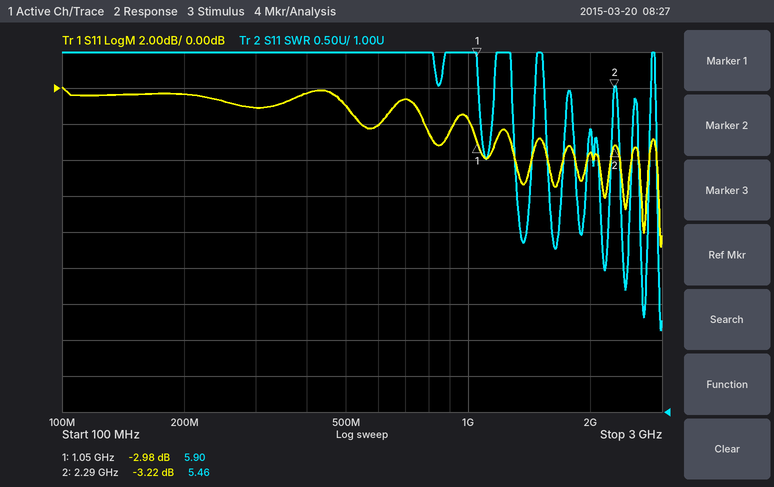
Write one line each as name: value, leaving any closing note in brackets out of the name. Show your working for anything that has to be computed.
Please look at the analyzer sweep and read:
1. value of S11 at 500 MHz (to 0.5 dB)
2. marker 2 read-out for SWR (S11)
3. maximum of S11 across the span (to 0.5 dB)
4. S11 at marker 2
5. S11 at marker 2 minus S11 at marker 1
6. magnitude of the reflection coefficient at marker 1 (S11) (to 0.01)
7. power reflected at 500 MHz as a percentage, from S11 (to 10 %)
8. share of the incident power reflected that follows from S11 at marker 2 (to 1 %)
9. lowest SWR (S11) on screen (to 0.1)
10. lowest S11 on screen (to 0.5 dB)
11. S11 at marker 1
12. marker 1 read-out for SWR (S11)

value of S11 at 500 MHz: -1.0 dB
marker 2 read-out for SWR: 5.46
maximum of S11 across the span: 0.0 dB
S11 at marker 2: -3.22 dB
S11 at marker 2 minus S11 at marker 1: -3.22 − (-2.98) = -0.24 dB
magnitude of the reflection coefficient at marker 1 (S11): 10^(-2.98/20) ≈ 0.71
power reflected at 500 MHz as a percentage, from S11: 10^(-1/10) ≈ 79.4 %, so 80 % to the nearest 10 %
share of the incident power reflected that follows from S11 at marker 2: 10^(-3.22/10) ≈ 48 %
lowest SWR (S11) on screen: 2.1
lowest S11 on screen: -9.0 dB
S11 at marker 1: -2.98 dB
marker 1 read-out for SWR: 5.90
